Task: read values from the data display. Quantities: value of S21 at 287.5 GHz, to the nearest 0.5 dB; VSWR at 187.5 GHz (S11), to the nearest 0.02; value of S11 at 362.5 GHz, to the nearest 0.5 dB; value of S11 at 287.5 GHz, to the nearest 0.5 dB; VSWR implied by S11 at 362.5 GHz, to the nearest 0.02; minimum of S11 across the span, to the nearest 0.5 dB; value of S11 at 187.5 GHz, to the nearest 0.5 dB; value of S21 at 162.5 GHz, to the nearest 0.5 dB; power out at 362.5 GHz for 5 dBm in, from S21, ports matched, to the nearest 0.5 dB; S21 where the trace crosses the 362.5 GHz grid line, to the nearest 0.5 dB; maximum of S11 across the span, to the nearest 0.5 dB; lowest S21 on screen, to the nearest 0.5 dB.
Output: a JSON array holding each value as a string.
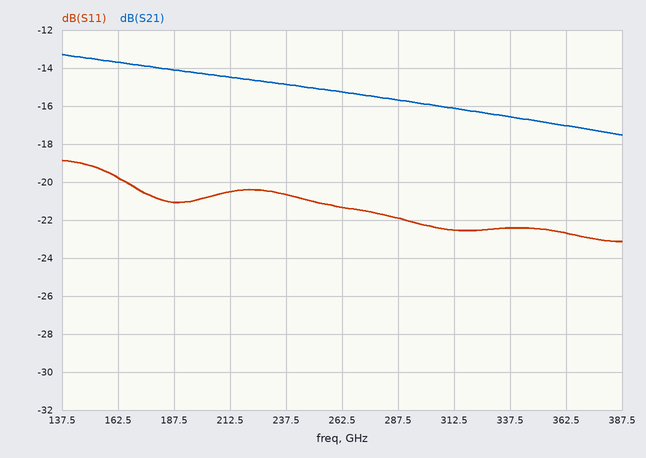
["-15.5 dB", "1.20", "-22.5 dB", "-22.0 dB", "1.16", "-23.0 dB", "-21.0 dB", "-13.5 dB", "-12.0 dBm", "-17.0 dB", "-19.0 dB", "-17.5 dB"]
